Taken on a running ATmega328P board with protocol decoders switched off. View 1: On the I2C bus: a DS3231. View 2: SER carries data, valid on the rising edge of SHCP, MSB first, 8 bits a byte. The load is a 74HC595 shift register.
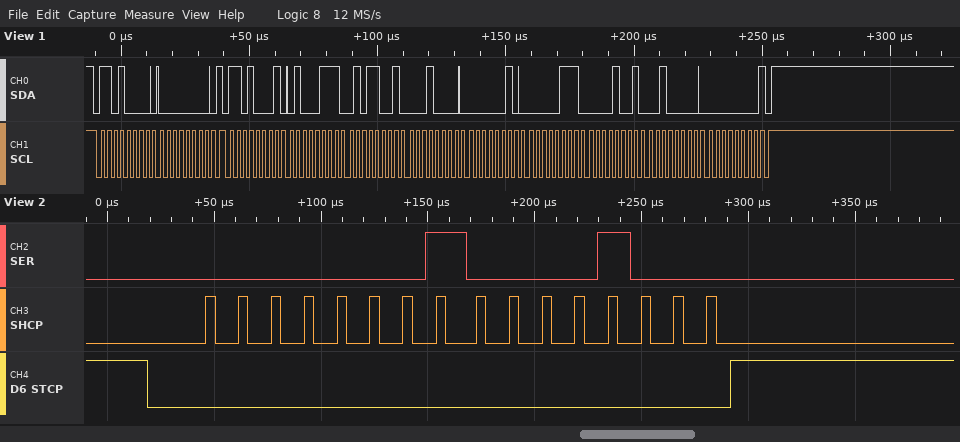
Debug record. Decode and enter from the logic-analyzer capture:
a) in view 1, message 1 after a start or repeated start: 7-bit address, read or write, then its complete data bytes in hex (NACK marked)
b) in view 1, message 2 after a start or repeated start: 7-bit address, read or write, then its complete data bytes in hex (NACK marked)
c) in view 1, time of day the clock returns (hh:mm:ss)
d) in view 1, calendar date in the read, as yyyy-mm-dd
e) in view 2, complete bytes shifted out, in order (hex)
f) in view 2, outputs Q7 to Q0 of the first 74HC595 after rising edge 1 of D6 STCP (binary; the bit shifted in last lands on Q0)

0x68 write: 00
0x68 read: 47 59 10 02 07 09 20 00 NACK
10:59:47
2020-09-07
01 08
00001000
